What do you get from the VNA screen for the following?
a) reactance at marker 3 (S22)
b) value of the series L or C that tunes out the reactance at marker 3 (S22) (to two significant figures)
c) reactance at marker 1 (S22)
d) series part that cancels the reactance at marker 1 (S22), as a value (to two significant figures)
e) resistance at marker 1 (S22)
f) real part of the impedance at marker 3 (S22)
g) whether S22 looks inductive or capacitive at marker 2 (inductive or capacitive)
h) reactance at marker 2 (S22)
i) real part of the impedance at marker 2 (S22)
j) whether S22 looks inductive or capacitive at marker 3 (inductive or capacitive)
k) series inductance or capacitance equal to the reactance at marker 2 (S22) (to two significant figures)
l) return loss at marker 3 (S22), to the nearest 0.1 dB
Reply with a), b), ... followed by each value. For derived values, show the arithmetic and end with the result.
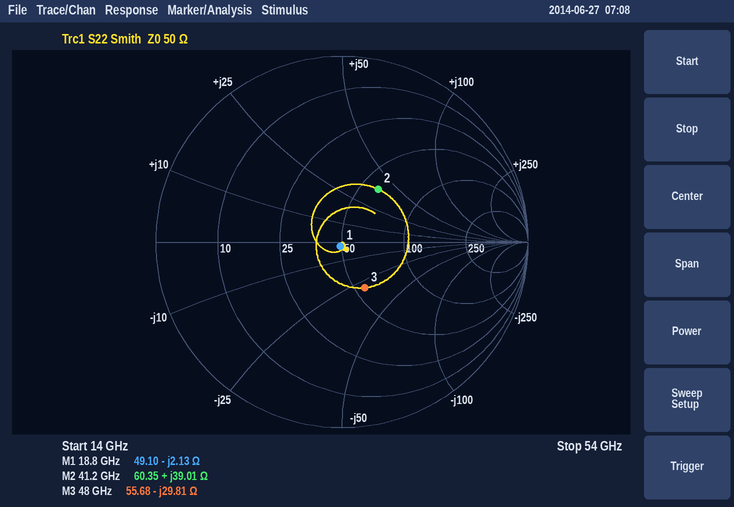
a) -29.81 Ω
b) L = 29.81 Ω/(2π × 48 GHz) ≈ 99 pH
c) -2.13 Ω
d) L = 2.13 Ω/(2π × 18.8 GHz) ≈ 18 pH
e) 49.10 Ω
f) 55.68 Ω
g) inductive
h) +39.01 Ω
i) 60.35 Ω
j) capacitive
k) L = 39.01 Ω/(2π × 41.2 GHz) ≈ 151 pH, so 150 pH to two significant figures
l) 11.2 dB
